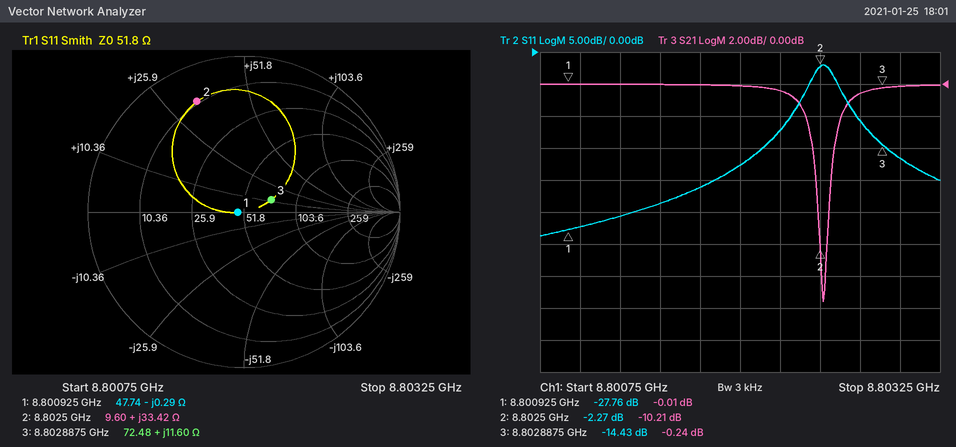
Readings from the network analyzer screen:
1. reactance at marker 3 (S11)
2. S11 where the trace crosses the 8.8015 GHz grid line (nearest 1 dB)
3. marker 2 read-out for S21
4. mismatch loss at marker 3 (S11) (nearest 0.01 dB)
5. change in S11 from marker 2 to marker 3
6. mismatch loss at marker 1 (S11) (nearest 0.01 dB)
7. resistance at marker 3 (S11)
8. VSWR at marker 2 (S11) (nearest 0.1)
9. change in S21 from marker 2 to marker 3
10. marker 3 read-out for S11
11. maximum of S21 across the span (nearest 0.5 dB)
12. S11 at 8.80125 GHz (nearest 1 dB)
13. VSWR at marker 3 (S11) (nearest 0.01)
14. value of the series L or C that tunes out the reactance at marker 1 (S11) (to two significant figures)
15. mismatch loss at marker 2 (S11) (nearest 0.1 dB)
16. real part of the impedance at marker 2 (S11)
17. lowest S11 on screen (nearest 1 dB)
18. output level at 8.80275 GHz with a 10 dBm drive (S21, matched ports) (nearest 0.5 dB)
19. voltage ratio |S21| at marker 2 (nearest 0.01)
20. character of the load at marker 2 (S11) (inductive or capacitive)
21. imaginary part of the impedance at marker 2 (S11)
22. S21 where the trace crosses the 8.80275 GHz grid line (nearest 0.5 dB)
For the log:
+11.60 Ω
-24 dB
-10.21 dB
0.16 dB
-12.16 dB
0.01 dB
72.48 Ω
7.7
9.97 dB
-14.43 dB
0.0 dB
-26 dB
1.47
5.2 pH
3.9 dB
9.60 Ω
-29 dB
9.5 dBm
0.31
inductive
+33.42 Ω
-0.5 dB
